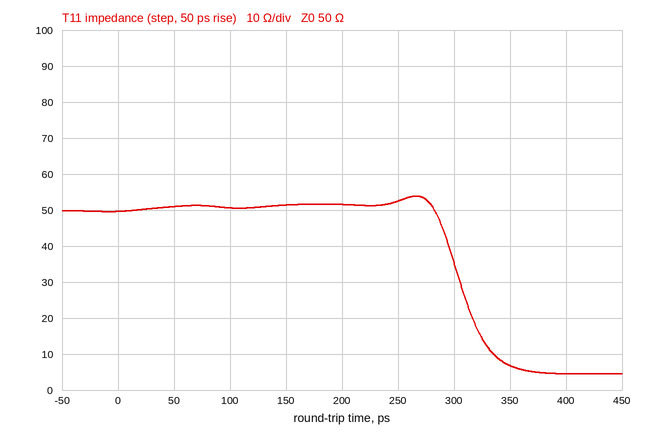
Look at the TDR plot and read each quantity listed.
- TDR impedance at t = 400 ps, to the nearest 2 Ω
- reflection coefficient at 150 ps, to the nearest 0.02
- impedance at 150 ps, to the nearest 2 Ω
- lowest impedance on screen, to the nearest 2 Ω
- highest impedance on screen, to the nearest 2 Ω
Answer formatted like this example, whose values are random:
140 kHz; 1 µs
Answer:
4 Ω; +0.02; 52 Ω; 4 Ω; 54 Ω
